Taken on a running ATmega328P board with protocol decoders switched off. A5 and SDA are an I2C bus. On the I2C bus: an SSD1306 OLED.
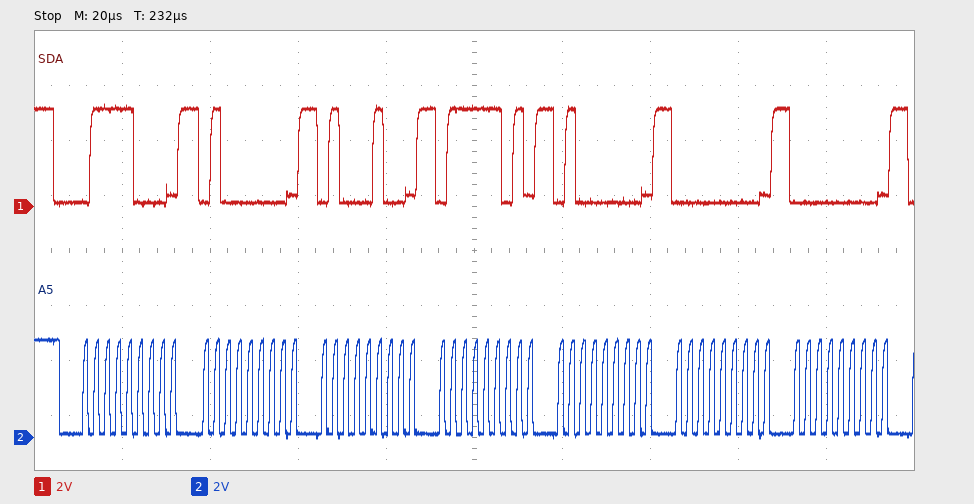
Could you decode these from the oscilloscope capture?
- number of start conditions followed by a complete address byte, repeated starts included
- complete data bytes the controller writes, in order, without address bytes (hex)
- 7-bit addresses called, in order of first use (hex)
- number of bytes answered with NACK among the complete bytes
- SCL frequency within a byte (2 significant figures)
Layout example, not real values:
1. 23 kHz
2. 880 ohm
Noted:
1. 1
2. 40 44 7D 40 00 00
3. 0x3C
4. 0
5. 400 kHz
